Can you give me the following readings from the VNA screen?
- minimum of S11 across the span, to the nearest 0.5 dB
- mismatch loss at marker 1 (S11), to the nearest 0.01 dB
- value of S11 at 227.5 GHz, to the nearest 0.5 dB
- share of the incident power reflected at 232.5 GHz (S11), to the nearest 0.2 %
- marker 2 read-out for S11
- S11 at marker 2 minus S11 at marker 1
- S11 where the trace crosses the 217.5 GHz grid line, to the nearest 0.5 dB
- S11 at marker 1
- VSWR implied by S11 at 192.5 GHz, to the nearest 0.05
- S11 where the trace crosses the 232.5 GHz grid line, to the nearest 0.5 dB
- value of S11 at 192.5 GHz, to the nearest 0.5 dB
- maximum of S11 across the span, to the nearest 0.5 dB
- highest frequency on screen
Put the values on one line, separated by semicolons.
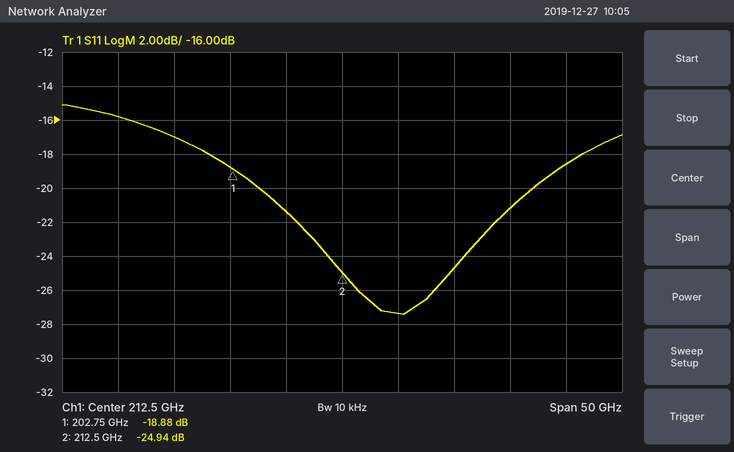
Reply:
-27.5 dB; 0.06 dB; -21.0 dB; 1.4 %; -24.94 dB; -6.06 dB; -27.5 dB; -18.88 dB; 1.40; -18.5 dB; -16.0 dB; -15.0 dB; 237.5 GHz
